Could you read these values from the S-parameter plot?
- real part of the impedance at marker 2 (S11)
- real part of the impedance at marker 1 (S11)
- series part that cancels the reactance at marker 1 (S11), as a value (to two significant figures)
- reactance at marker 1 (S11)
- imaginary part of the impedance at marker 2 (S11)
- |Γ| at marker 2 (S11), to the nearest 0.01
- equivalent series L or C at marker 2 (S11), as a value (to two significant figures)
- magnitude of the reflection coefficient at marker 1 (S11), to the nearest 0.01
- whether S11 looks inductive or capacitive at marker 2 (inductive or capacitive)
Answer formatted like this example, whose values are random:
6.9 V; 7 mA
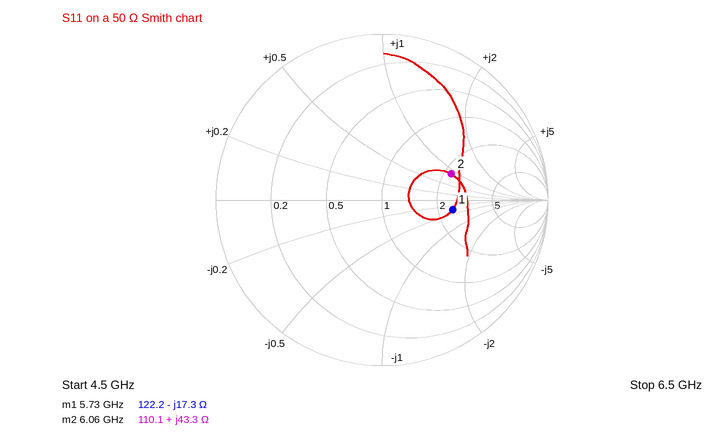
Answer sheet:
110.1 Ω; 122.2 Ω; 480 pH; -17.3 Ω; +43.3 Ω; 0.45; 1.1 nH; 0.43; inductive
